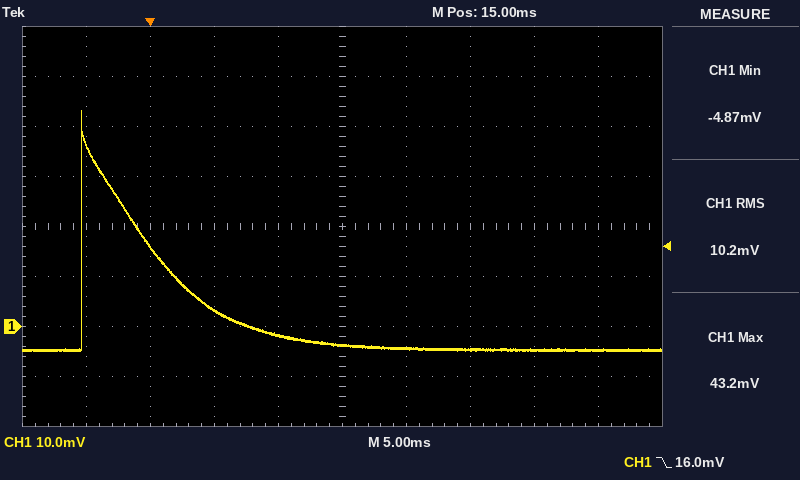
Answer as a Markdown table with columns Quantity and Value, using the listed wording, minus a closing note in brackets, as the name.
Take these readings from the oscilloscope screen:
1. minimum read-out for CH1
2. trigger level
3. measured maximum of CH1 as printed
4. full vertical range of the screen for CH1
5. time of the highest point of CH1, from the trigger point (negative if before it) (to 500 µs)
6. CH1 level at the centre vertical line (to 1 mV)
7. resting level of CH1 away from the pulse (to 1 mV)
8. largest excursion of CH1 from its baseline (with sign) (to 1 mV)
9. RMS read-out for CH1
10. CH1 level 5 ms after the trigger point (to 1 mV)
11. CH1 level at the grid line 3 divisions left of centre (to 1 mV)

| Quantity | Value |
|---|---|
| minimum read-out for CH1 | -4.87 mV |
| trigger level | 16.0 mV |
| measured maximum of CH1 as printed | 43.2 mV |
| full vertical range of the screen for CH1 | 80 mV |
| time of the highest point of CH1, from the trigger point (negative if before it) | -5.5 ms |
| CH1 level at the centre vertical line | -4 mV |
| resting level of CH1 away from the pulse | -5 mV |
| largest excursion of CH1 from its baseline (with sign) | +48 mV |
| RMS read-out for CH1 | 10.2 mV |
| CH1 level 5 ms after the trigger point | 3 mV |
| CH1 level at the grid line 3 divisions left of centre | 16 mV |
